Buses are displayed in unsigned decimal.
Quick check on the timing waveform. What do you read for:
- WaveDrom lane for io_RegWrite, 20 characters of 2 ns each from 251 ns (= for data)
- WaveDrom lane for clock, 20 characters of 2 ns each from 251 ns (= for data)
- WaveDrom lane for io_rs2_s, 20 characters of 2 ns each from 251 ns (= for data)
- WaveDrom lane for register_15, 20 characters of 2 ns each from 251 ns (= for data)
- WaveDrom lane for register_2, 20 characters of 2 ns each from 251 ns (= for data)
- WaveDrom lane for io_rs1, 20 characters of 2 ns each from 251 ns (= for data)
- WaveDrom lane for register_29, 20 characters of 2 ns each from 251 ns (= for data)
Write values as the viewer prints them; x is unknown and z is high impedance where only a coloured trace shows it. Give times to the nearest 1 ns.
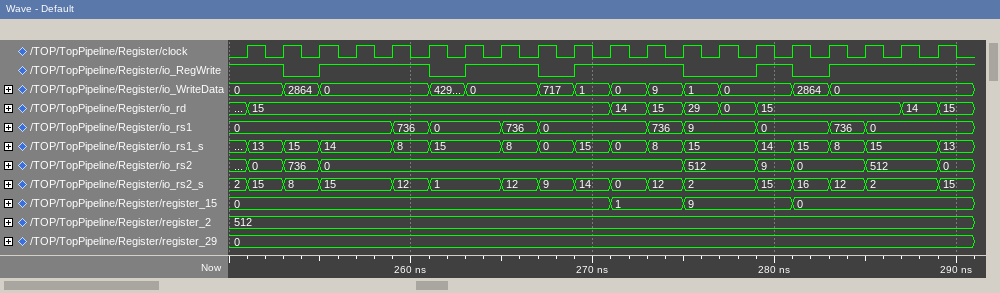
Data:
{name: 'io_RegWrite', wave: '101..01.01..0.101...'}
{name: 'clock', wave: 'p...................'}
{name: 'io_rs2_s', wave: '===.==.======.====.=', data: '15 8 15 12 1 12 9 14 0 12 2 15 16 12 2 15'}
{name: 'register_15', wave: '=.........=.=..=....', data: '0 1 9 0'}
{name: 'register_2', wave: '=...................', data: '512'}
{name: 'io_rs1', wave: '=...==.==..==.=.==..', data: '0 736 0 736 0 736 9 0 736 0'}
{name: 'register_29', wave: '=...................', data: '0'}
